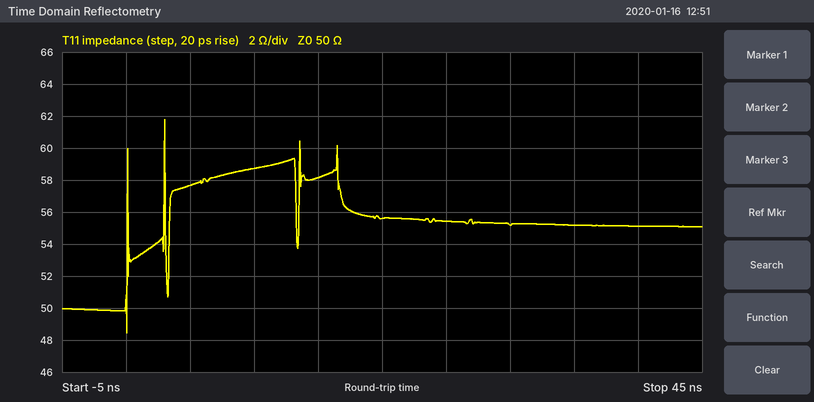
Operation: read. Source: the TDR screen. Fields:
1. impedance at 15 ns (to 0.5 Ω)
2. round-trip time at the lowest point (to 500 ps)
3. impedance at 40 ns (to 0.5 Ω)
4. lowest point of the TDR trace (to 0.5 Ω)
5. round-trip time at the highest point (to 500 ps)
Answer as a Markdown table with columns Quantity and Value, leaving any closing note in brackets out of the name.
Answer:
| Quantity | Value |
|---|---|
| impedance at 15 ns | 58.0 Ω |
| round-trip time at the lowest point | 0.0 ns |
| impedance at 40 ns | 55.0 Ω |
| lowest point of the TDR trace | 48.5 Ω |
| round-trip time at the highest point | 3.0 ns |
